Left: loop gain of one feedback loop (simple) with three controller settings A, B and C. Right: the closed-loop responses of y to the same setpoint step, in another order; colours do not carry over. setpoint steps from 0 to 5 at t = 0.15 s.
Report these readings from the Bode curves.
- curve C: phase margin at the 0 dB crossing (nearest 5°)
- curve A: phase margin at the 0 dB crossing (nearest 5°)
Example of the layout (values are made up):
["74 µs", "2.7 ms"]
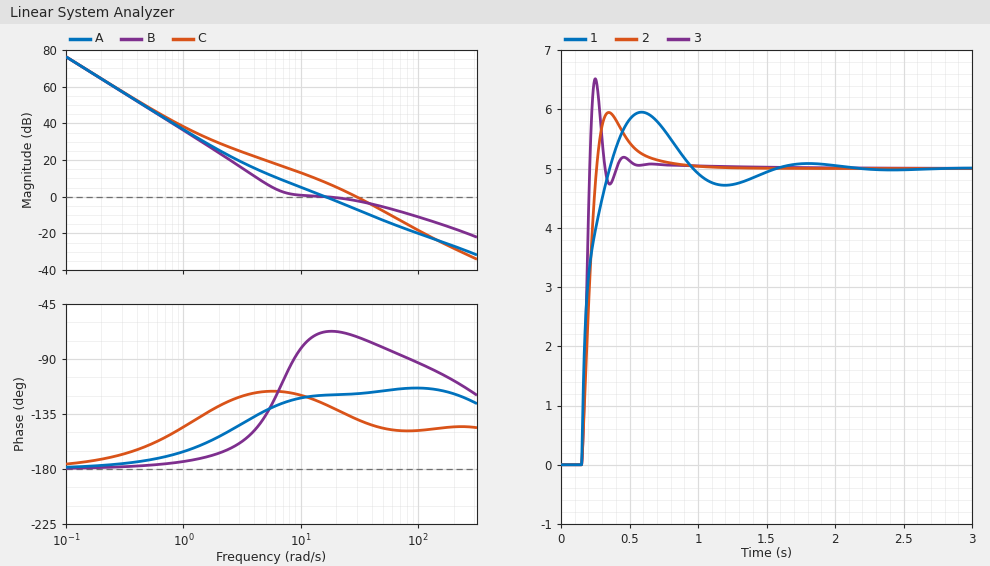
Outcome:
["40°", "60°"]
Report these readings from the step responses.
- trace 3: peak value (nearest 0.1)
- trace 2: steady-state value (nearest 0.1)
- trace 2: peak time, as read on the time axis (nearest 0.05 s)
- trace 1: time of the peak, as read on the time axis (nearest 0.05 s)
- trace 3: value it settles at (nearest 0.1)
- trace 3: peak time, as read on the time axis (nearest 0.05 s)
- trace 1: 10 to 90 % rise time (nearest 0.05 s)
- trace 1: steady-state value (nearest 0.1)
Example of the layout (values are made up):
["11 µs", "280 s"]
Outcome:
["6.5", "5.0", "0.35 s", "0.60 s", "5.0", "0.25 s", "0.15 s", "5.0"]
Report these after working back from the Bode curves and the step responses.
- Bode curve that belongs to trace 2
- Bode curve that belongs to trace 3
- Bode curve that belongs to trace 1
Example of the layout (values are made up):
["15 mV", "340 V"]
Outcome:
["A", "C", "B"]
